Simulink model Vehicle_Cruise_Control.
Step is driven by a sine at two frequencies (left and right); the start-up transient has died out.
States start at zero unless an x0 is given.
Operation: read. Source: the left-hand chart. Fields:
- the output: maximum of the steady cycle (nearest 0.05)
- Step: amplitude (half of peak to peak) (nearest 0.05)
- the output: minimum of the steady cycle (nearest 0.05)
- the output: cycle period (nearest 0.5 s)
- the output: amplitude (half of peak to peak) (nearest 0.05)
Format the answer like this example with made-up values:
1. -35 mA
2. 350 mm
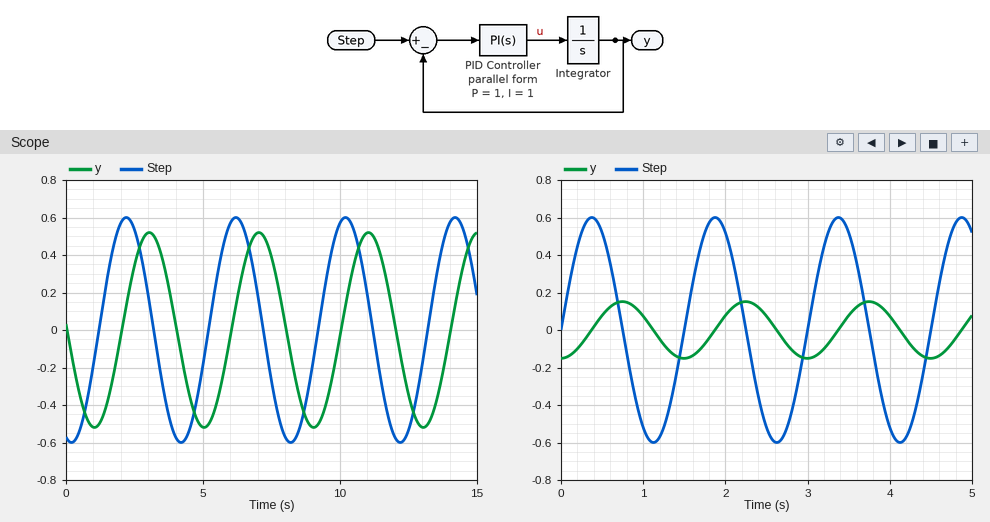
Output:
1. 0.50
2. 0.60
3. -0.50
4. 4.0 s
5. 0.50
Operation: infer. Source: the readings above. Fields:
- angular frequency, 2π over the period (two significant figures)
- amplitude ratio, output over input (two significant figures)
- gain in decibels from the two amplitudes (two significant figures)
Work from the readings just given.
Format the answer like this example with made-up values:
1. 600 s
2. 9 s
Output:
1. 1.6 rad/s
2. 0.83
3. -1.6 dB
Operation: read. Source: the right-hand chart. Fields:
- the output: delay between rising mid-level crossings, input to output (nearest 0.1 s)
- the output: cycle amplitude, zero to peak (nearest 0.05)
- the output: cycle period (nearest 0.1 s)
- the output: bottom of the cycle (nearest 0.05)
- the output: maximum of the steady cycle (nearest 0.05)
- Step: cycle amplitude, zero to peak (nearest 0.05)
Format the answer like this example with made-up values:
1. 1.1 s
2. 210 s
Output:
1. 0.4 s
2. 0.15
3. 1.5 s
4. -0.15
5. 0.15
6. 0.60
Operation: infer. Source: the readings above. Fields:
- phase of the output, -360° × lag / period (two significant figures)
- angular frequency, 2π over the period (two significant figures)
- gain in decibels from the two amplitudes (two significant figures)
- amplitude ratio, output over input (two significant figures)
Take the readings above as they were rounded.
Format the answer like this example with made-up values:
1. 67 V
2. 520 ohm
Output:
1. -96°
2. 4.2 rad/s
3. -12 dB
4. 0.25
